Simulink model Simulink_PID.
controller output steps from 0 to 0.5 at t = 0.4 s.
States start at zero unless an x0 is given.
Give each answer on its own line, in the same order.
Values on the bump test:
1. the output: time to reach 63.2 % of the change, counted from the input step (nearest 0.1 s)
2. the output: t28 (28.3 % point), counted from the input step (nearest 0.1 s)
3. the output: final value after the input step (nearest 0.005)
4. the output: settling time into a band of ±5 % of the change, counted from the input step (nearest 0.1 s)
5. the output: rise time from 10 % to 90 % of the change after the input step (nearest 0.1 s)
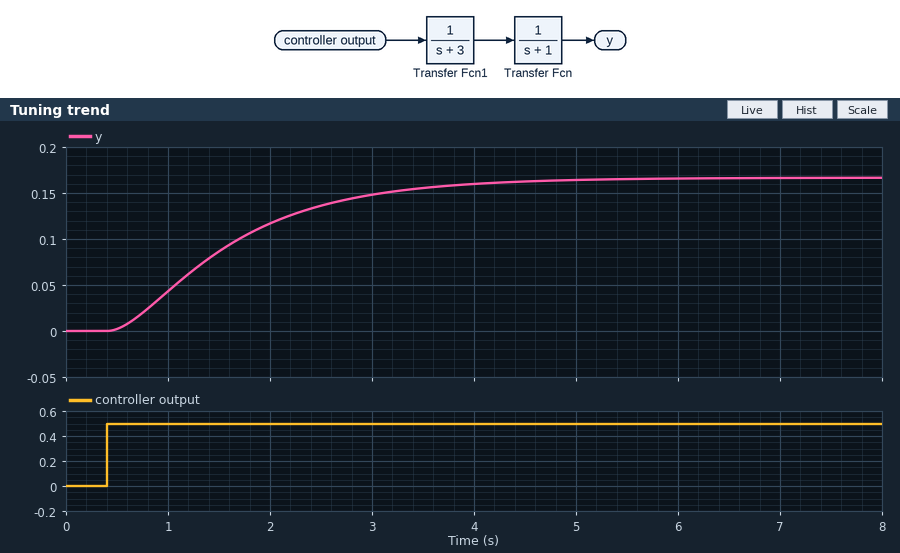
1.4 s
0.6 s
0.165
3.4 s
2.4 s
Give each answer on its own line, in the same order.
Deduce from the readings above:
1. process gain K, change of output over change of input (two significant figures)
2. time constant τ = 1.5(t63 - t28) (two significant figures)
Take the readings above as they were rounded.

0.33
1.2 s
